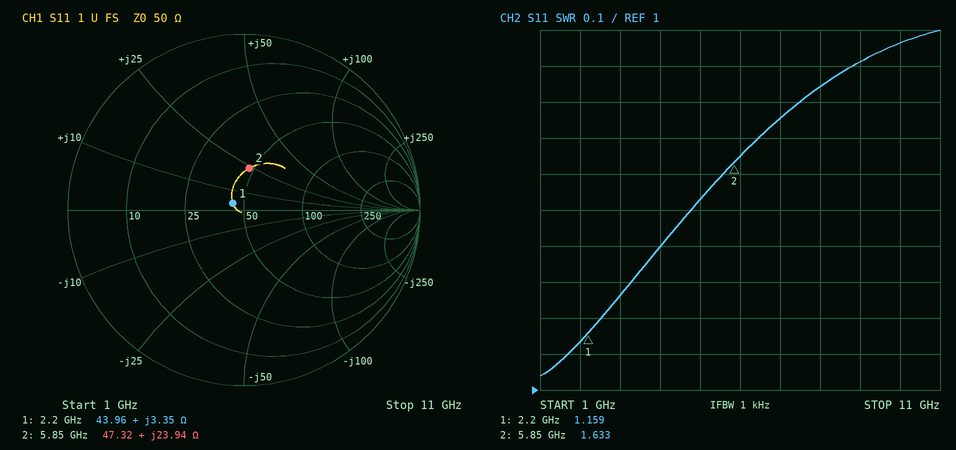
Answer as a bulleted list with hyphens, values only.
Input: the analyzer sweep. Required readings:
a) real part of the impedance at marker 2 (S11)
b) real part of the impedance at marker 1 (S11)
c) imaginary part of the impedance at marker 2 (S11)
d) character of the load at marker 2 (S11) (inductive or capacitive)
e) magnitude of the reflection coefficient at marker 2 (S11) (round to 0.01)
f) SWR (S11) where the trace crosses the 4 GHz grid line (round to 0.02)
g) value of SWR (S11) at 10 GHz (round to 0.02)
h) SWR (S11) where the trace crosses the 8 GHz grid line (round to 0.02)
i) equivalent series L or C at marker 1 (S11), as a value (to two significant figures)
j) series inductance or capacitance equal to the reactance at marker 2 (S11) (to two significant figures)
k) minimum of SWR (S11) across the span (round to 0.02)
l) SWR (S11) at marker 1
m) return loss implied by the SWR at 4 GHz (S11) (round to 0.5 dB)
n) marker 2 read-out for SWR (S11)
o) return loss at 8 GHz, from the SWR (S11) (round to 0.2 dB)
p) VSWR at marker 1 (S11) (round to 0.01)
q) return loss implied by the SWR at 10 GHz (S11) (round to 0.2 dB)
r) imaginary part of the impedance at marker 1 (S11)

- 47.32 Ω
- 43.96 Ω
- +23.94 Ω
- inductive
- 0.24
- 1.40
- 1.96
- 1.84
- 240 pH
- 650 pH
- 1.04
- 1.159
- 15.5 dB
- 1.633
- 10.6 dB
- 1.16
- 9.8 dB
- +3.35 Ω
